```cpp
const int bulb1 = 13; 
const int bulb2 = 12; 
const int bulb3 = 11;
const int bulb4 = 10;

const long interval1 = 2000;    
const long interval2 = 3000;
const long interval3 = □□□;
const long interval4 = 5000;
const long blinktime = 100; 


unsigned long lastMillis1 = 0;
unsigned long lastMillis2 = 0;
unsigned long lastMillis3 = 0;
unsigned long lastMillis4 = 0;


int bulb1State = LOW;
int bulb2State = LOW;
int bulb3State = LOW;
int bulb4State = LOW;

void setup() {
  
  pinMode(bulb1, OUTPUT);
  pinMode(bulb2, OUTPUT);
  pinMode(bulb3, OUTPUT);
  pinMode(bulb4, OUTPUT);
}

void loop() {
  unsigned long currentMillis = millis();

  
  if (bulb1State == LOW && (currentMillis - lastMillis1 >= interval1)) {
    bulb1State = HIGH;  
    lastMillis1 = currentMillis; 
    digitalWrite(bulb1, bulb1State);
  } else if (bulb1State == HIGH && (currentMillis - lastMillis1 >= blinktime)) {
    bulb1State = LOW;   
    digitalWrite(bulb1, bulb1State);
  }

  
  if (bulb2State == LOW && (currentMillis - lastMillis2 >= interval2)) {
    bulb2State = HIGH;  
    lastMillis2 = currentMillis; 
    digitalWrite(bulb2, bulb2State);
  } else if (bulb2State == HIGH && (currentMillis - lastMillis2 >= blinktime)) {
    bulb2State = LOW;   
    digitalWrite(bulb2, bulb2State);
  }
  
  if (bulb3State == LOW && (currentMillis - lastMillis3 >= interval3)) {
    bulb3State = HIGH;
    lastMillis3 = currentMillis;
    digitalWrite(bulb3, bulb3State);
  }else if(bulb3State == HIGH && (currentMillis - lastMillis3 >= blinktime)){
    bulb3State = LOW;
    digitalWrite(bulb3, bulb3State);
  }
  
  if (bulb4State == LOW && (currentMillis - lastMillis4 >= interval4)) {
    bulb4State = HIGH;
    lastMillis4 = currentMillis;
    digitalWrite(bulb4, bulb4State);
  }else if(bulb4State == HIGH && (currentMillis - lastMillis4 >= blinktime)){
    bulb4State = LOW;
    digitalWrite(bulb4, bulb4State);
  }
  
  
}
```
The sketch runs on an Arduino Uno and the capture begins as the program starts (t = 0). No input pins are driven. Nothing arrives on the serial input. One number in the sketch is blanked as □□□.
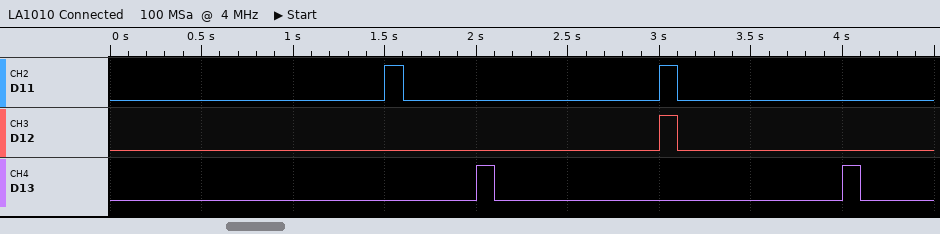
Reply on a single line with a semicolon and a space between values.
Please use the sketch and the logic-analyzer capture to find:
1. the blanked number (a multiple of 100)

1500
